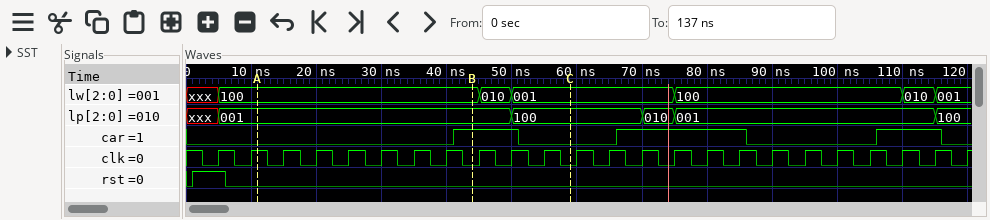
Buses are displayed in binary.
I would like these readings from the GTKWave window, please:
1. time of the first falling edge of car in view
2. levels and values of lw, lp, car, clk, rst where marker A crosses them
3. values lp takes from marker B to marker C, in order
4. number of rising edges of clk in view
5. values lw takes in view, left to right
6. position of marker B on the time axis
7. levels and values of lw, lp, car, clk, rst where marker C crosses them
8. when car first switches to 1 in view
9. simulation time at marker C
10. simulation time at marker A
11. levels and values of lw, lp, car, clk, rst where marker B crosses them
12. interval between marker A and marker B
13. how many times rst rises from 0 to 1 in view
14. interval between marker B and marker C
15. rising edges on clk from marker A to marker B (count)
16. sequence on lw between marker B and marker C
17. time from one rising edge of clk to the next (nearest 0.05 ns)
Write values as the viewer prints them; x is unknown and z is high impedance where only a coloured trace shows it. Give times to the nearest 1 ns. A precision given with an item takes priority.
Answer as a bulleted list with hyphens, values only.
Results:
- 51 ns
- lw=100, lp=001, car=0, clk=1, rst=0
- 001, 100
- 24
- xxx, 100, 010, 001, 100, 010, 001
- 44 ns
- lw=001, lp=100, car=0, clk=0, rst=0
- 41 ns
- 59 ns
- 11 ns
- lw=100, lp=001, car=1, clk=0, rst=0
- 33 ns
- 1
- 15 ns
- 6
- 100, 010, 001
- 5 ns
